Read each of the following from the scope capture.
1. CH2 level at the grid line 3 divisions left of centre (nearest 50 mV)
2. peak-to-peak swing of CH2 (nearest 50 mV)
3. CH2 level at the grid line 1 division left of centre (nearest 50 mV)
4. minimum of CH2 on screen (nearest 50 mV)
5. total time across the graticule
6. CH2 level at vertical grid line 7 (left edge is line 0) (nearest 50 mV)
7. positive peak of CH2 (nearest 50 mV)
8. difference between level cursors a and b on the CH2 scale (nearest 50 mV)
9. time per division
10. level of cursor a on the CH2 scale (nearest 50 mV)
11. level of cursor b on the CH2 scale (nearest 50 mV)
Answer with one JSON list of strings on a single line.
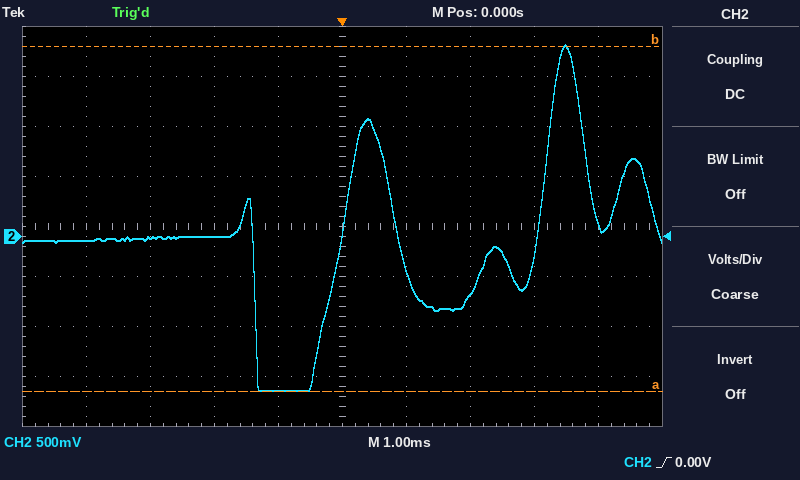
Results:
["0 mV", "3.45 V", "-1.55 V", "-1.55 V", "10 ms", "-600 mV", "1.90 V", "3.45 V", "1 ms", "-1.55 V", "1.90 V"]
